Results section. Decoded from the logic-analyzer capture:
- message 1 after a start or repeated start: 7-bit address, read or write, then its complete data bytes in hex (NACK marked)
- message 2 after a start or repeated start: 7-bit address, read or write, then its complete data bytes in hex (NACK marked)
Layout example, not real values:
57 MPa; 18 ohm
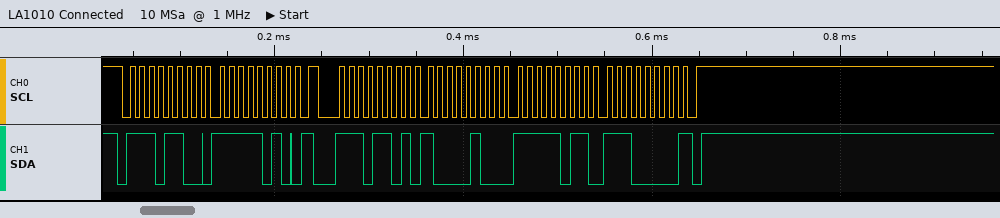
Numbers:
0x76 write: FA; 0x76 read: 84 FB E0 NACK
